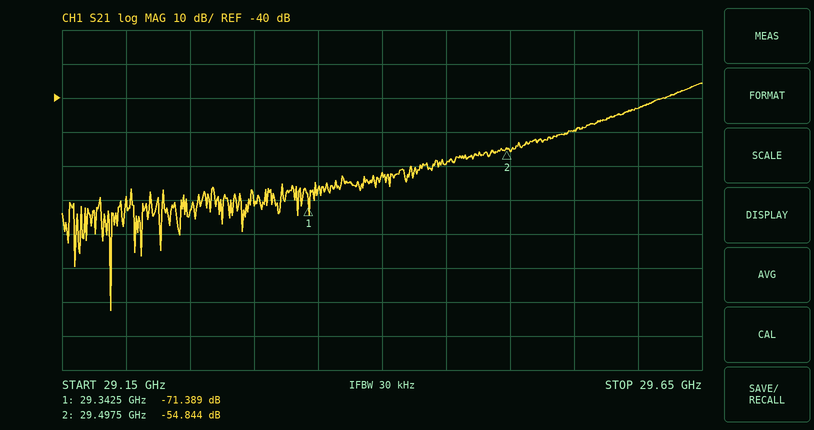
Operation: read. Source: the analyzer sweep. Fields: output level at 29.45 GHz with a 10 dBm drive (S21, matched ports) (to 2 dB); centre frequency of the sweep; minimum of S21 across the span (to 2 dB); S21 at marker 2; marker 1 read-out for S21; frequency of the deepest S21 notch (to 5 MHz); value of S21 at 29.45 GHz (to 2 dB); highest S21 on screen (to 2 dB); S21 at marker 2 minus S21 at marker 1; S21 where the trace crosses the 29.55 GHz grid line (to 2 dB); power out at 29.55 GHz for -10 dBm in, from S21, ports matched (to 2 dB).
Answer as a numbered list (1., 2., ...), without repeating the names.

1. -50 dBm
2. 29.4 GHz
3. -102 dB
4. -54.844 dB
5. -71.389 dB
6. 29.190 GHz
7. -60 dB
8. -36 dB
9. 16.545 dB
10. -50 dB
11. -60 dBm
